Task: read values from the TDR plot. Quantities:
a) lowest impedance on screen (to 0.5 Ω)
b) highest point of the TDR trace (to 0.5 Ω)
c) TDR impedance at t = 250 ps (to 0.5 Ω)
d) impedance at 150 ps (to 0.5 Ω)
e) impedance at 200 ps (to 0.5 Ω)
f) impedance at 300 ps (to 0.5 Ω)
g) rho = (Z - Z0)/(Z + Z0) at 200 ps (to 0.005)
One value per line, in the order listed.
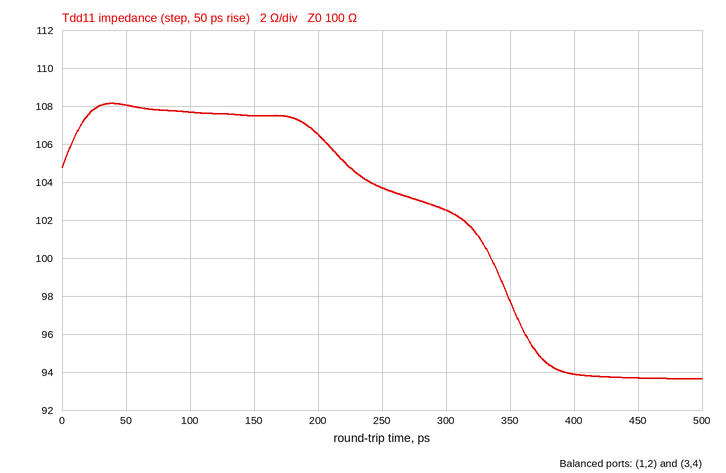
93.5 Ω
108.0 Ω
103.5 Ω
107.5 Ω
106.5 Ω
102.5 Ω
+0.030
